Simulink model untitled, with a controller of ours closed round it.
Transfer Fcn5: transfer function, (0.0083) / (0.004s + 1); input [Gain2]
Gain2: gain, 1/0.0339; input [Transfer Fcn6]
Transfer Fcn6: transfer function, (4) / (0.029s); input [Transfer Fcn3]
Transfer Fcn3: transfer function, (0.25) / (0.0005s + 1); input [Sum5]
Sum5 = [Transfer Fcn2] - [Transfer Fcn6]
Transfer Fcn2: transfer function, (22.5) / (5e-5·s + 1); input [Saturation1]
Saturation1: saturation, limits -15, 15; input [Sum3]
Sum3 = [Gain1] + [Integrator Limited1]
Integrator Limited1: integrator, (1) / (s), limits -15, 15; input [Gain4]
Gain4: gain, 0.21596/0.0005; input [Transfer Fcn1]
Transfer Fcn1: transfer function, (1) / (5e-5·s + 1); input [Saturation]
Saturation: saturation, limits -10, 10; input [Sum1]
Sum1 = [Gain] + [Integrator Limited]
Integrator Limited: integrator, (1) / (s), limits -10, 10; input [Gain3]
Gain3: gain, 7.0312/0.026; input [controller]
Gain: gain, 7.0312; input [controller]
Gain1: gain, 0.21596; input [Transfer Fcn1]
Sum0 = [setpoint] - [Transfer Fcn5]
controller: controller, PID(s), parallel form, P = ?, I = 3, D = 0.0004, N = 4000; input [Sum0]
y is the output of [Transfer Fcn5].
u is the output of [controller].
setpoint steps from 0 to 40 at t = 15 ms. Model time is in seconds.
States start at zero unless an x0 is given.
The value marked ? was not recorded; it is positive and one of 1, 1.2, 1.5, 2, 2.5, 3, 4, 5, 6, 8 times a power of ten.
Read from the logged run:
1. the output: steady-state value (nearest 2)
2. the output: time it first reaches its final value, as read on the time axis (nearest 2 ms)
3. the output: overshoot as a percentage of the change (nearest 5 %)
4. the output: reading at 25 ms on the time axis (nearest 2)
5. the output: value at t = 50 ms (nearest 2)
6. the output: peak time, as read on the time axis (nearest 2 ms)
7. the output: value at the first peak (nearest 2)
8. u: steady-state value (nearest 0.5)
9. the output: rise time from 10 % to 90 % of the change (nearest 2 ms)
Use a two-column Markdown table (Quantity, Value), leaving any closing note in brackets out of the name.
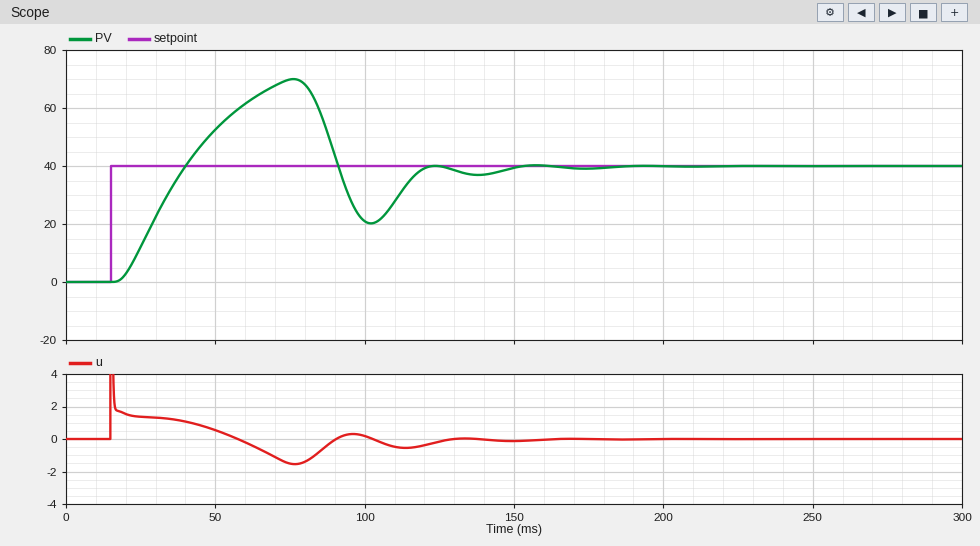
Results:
| Quantity | Value |
|---|---|
| the output: steady-state value | 40 |
| the output: time it first reaches its final value, as read on the time axis | 40 ms |
| the output: overshoot as a percentage of the change | 75 % |
| the output: reading at 25 ms on the time axis | 12 |
| the output: value at t = 50 ms | 52 |
| the output: peak time, as read on the time axis | 76 ms |
| the output: value at the first peak | 70 |
| u: steady-state value | 0.0 |
| the output: rise time from 10 % to 90 % of the change | 16 ms |
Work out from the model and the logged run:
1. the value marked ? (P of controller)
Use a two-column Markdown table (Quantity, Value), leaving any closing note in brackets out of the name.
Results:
| Quantity | Value |
|---|---|
| the value marked ? | 0.04 |
